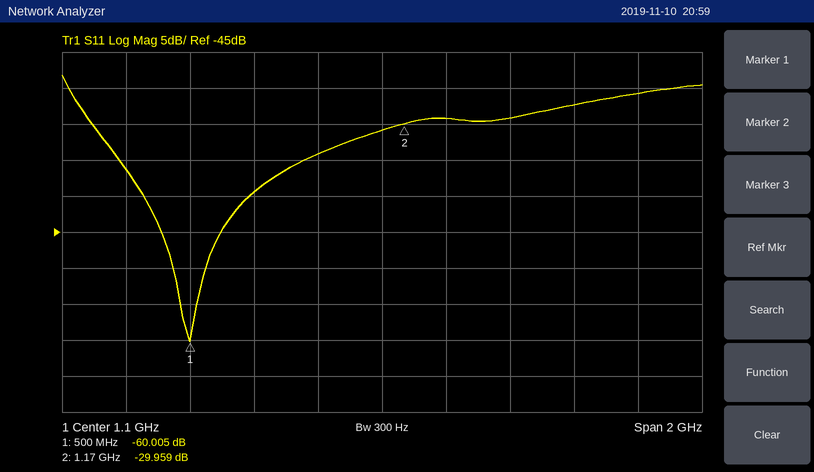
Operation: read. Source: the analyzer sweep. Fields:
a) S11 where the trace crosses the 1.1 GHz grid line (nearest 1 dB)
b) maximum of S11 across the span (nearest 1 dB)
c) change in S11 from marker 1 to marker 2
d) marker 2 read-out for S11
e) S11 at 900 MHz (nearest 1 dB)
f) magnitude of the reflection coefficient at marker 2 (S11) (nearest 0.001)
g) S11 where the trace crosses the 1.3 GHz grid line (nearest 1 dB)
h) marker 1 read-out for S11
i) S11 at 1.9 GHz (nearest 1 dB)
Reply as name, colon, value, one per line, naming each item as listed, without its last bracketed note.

S11 where the trace crosses the 1.1 GHz grid line: -31 dB
maximum of S11 across the span: -23 dB
change in S11 from marker 1 to marker 2: 30.046 dB
marker 2 read-out for S11: -29.959 dB
S11 at 900 MHz: -34 dB
magnitude of the reflection coefficient at marker 2 (S11): 0.032
S11 where the trace crosses the 1.3 GHz grid line: -29 dB
marker 1 read-out for S11: -60.005 dB
S11 at 1.9 GHz: -26 dB
